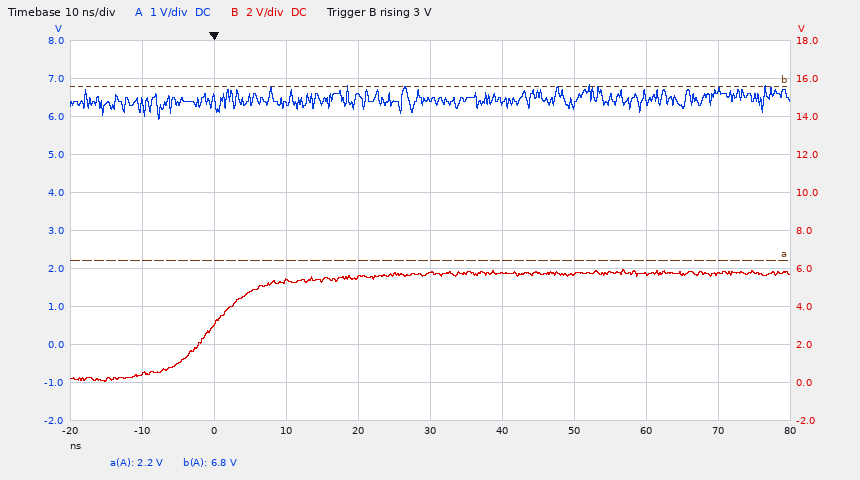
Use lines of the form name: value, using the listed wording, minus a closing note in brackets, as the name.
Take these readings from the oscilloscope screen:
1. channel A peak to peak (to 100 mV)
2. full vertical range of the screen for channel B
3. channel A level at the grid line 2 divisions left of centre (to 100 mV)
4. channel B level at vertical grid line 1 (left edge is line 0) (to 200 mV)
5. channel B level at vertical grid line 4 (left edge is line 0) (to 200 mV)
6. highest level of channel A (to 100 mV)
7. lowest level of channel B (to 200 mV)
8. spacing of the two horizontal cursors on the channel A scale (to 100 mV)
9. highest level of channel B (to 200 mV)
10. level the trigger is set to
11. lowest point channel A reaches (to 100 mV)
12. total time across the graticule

channel A peak to peak: 900 mV
full vertical range of the screen for channel B: 20 V
channel A level at the grid line 2 divisions left of centre: 6.3 V
channel B level at vertical grid line 1 (left edge is line 0): 400 mV
channel B level at vertical grid line 4 (left edge is line 0): 5.6 V
highest level of channel A: 6.8 V
lowest level of channel B: 0.0 V
spacing of the two horizontal cursors on the channel A scale: 4.6 V
highest level of channel B: 6.0 V
level the trigger is set to: 3 V
lowest point channel A reaches: 5.9 V
total time across the graticule: 100 ns
